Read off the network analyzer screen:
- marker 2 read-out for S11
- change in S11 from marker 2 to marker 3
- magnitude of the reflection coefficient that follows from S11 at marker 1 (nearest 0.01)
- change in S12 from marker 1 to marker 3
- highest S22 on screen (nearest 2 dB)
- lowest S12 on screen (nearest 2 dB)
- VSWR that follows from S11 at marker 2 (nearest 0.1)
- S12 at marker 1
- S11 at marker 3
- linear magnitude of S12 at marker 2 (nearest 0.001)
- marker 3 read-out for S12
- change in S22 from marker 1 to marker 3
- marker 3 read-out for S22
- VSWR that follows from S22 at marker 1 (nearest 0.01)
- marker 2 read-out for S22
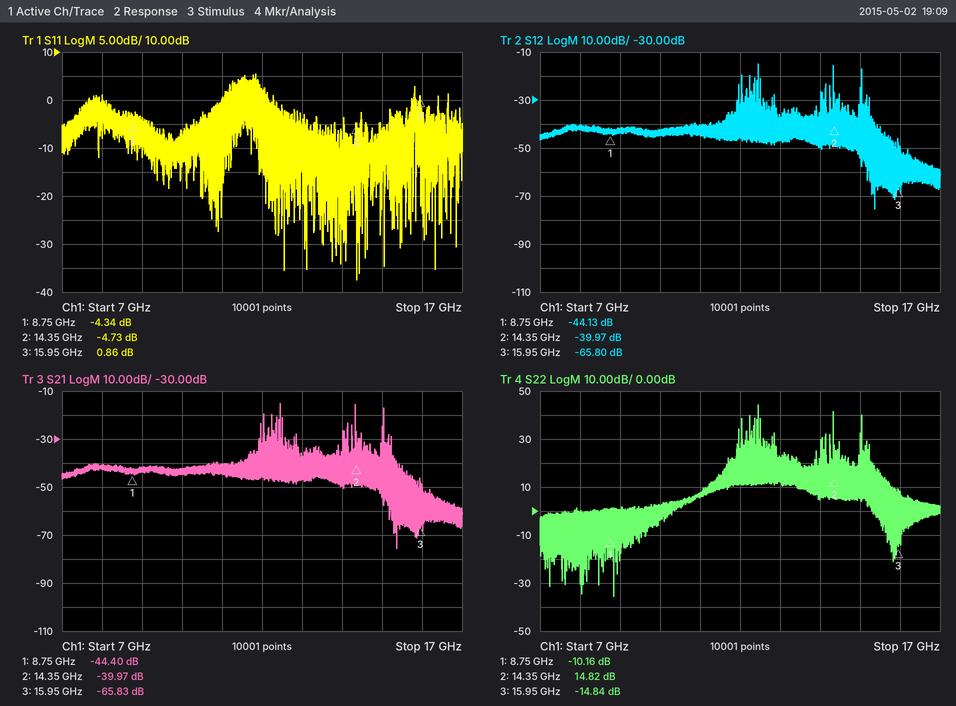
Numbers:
-4.73 dB
5.59 dB
0.61
-21.67 dB
44 dB
-76 dB
3.8
-44.13 dB
0.86 dB
0.010
-65.80 dB
-4.68 dB
-14.84 dB
1.90
14.82 dB
